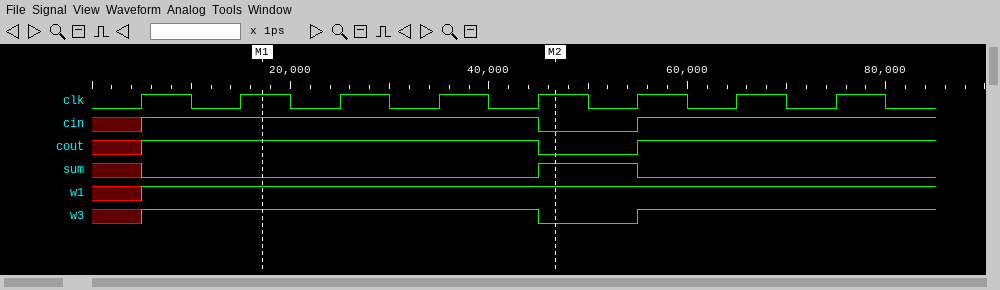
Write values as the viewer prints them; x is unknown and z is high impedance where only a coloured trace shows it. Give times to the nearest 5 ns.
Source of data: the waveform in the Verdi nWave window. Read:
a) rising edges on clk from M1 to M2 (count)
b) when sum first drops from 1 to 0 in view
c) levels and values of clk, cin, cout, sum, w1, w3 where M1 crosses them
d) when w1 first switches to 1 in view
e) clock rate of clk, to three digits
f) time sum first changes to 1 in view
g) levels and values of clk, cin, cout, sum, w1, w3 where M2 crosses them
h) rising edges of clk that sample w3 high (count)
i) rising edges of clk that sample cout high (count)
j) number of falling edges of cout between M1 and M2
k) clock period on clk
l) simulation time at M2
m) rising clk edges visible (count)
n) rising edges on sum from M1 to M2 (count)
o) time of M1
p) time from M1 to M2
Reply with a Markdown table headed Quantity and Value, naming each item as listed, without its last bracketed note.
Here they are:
| Quantity | Value |
|---|---|
| rising edges on clk from M1 to M2 | 3 |
| when sum first drops from 1 to 0 in view | 55 ns |
| levels and values of clk, cin, cout, sum, w1, w3 where M1 crosses them | clk=1, cin=1, cout=1, sum=0, w1=1, w3=1 |
| when w1 first switches to 1 in view | 5 ns |
| clock rate of clk, to three digits | 100 MHz |
| time sum first changes to 1 in view | 45 ns |
| levels and values of clk, cin, cout, sum, w1, w3 where M2 crosses them | clk=1, cin=0, cout=0, sum=1, w1=1, w3=0 |
| rising edges of clk that sample w3 high | 6 |
| rising edges of clk that sample cout high | 6 |
| number of falling edges of cout between M1 and M2 | 1 |
| clock period on clk | 10 ns |
| simulation time at M2 | 45 ns |
| rising clk edges visible | 8 |
| rising edges on sum from M1 to M2 | 1 |
| time of M1 | 15 ns |
| time from M1 to M2 | 30 ns |
